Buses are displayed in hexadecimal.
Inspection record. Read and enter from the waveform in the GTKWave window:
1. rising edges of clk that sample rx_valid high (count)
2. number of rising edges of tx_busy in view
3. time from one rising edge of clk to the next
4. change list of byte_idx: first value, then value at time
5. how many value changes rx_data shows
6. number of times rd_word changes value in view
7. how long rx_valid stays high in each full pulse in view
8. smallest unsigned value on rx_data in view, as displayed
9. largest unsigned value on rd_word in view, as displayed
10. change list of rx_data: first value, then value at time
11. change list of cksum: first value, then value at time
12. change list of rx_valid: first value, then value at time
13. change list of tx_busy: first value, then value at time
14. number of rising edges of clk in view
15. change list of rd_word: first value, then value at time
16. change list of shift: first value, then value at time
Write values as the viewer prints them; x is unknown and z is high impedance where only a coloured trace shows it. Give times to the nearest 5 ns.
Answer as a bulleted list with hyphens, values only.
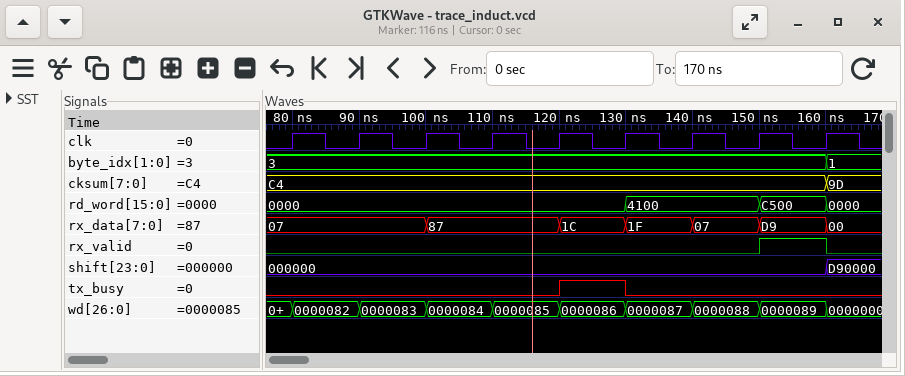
- 1
- 1
- 10 ns
- 3, 1 at 160 ns
- 6
- 3
- 10 ns
- 00
- C500
- 07, 87 at 100 ns, 1C at 120 ns, 1F at 130 ns, 07 at 140 ns, D9 at 150 ns, 00 at 160 ns
- C4, 9D at 160 ns
- 0, 1 at 150 ns, 0 at 160 ns
- 0, 1 at 120 ns, 0 at 130 ns
- 9
- 0000, 4100 at 130 ns, C500 at 150 ns, 0000 at 160 ns
- 000000, D90000 at 160 ns
